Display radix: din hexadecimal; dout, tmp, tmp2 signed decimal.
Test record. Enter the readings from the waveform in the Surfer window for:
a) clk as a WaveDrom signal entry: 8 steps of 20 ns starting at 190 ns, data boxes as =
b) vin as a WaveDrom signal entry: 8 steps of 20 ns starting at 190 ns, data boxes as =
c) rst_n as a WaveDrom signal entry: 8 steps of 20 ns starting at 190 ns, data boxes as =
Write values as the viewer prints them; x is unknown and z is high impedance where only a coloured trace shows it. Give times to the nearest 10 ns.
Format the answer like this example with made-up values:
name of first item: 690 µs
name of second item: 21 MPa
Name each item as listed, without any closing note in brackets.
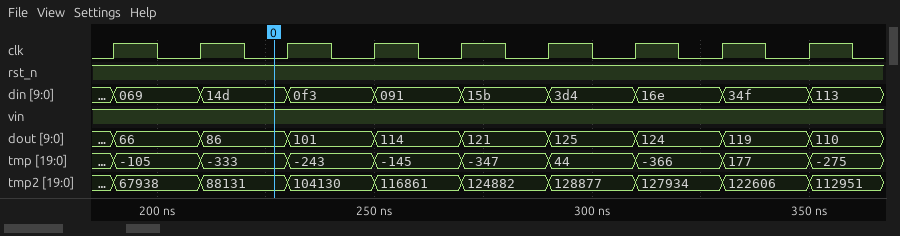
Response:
clk as a WaveDrom signal entry: 8 steps of 20 ns starting at 190 ns, data boxes as =: {name: 'clk', wave: 'p.......'}
vin as a WaveDrom signal entry: 8 steps of 20 ns starting at 190 ns, data boxes as =: {name: 'vin', wave: '1.......'}
rst_n as a WaveDrom signal entry: 8 steps of 20 ns starting at 190 ns, data boxes as =: {name: 'rst_n', wave: '1.......'}
